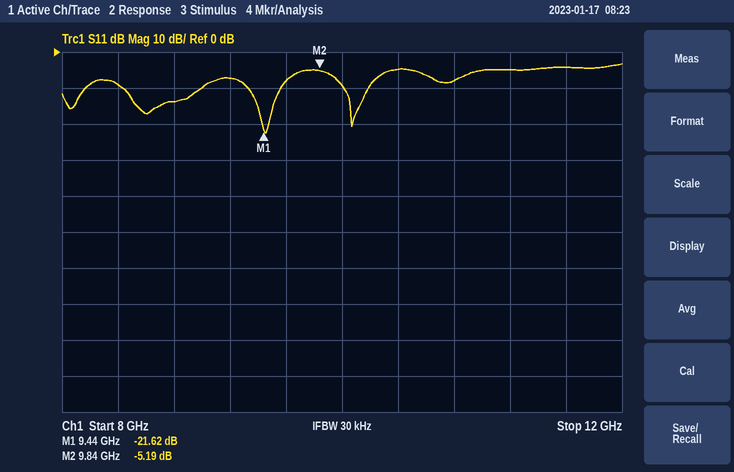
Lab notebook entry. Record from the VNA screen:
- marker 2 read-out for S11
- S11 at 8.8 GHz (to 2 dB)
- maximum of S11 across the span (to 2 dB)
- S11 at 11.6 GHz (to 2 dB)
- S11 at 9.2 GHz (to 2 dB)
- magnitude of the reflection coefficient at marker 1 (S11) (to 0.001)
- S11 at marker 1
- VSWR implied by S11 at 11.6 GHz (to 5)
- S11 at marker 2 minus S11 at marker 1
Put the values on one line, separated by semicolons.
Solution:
-5.19 dB; -14 dB; -4 dB; -4 dB; -8 dB; 0.083; -21.62 dB; 5; 16.43 dB
